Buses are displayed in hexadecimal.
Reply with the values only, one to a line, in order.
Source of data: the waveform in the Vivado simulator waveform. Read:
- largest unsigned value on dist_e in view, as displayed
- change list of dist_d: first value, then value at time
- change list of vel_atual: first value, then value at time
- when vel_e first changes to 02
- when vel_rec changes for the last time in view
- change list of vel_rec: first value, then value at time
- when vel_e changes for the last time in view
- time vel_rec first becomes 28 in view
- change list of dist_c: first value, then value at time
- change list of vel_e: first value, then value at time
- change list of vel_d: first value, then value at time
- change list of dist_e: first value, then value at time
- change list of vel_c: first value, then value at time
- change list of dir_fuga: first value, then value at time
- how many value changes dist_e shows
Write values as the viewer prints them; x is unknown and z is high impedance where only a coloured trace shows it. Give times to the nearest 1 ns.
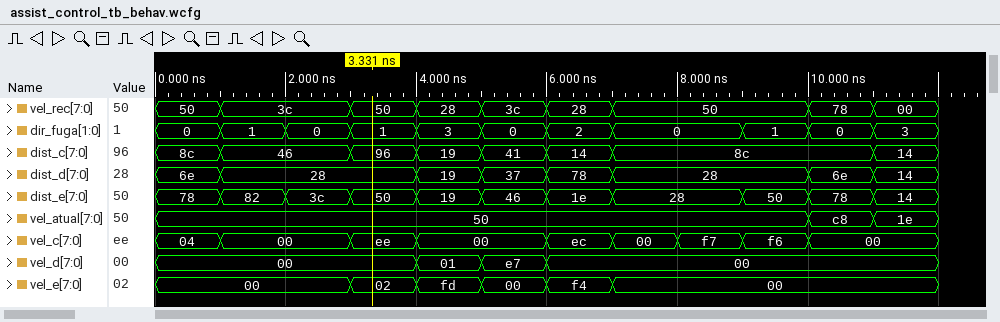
82
6e, 28 at 1 ns, 19 at 4 ns, 37 at 5 ns, 78 at 6 ns, 28 at 7 ns, 6e at 10 ns, 14 at 11 ns
50, c8 at 10 ns, 1e at 11 ns
3 ns
11 ns
50, 3c at 1 ns, 50 at 3 ns, 28 at 4 ns, 3c at 5 ns, 28 at 6 ns, 50 at 7 ns, 78 at 10 ns, 00 at 11 ns
7 ns
4 ns
8c, 46 at 1 ns, 96 at 3 ns, 19 at 4 ns, 41 at 5 ns, 14 at 6 ns, 8c at 7 ns, 14 at 11 ns
00, 02 at 3 ns, fd at 4 ns, 00 at 5 ns, f4 at 6 ns, 00 at 7 ns
00, 01 at 4 ns, e7 at 5 ns, 00 at 6 ns
78, 82 at 1 ns, 3c at 2 ns, 50 at 3 ns, 19 at 4 ns, 46 at 5 ns, 1e at 6 ns, 28 at 7 ns, 50 at 9 ns, 78 at 10 ns, 14 at 11 ns
04, 00 at 1 ns, ee at 3 ns, 00 at 4 ns, ec at 6 ns, 00 at 7 ns, f7 at 8 ns, f6 at 9 ns, 00 at 10 ns
0, 1 at 1 ns, 0 at 2 ns, 1 at 3 ns, 3 at 4 ns, 0 at 5 ns, 2 at 6 ns, 0 at 7 ns, 1 at 9 ns, 0 at 10 ns, 3 at 11 ns
10
